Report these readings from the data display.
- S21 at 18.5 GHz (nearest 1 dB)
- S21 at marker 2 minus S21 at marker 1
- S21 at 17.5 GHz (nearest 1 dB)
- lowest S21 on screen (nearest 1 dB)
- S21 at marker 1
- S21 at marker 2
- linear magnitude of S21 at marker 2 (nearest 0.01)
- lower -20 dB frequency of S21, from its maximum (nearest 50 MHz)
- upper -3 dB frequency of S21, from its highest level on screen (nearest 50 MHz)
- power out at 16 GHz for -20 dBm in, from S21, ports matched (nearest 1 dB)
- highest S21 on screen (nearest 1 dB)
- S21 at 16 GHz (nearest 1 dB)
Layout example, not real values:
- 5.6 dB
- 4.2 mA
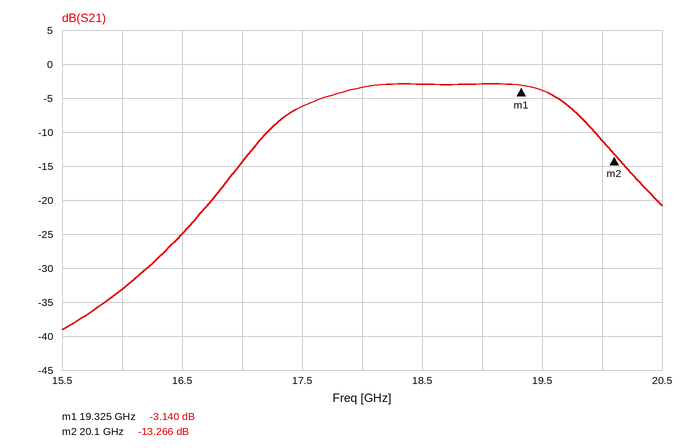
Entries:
- -3 dB
- -10.126 dB
- -6 dB
- -39 dB
- -3.140 dB
- -13.266 dB
- 0.22
- 16.60 GHz
- 19.70 GHz
- -53 dBm
- -3 dB
- -33 dB
